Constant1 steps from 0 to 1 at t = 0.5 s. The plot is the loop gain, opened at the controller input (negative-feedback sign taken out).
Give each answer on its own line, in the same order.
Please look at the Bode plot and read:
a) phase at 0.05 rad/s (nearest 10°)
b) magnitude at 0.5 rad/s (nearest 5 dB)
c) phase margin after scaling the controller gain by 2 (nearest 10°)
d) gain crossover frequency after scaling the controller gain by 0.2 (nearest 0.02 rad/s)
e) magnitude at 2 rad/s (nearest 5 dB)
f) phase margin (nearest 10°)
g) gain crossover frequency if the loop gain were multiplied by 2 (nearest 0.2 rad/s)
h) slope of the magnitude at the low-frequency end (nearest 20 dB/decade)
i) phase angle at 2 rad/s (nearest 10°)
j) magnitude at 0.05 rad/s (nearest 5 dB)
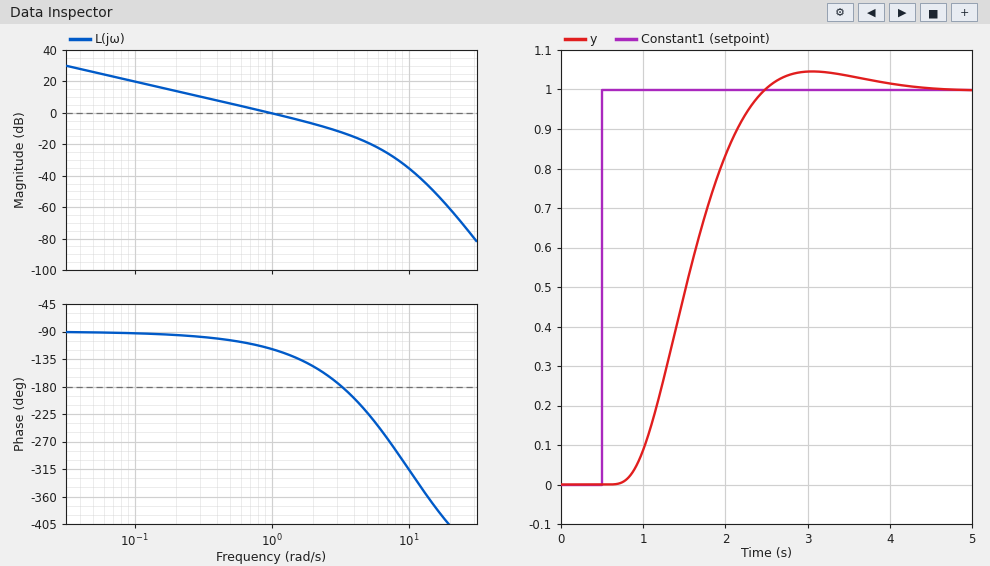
-90°
5 dB
40°
0.20 rad/s
-5 dB
60°
1.8 rad/s
-20 dB/decade
-150°
25 dB
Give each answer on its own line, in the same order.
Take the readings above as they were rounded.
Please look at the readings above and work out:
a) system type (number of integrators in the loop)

1
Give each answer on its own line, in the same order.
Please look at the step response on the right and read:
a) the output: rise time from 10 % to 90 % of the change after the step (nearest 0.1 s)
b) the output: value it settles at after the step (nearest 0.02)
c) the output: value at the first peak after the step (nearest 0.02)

1.1 s
1.00
1.04
